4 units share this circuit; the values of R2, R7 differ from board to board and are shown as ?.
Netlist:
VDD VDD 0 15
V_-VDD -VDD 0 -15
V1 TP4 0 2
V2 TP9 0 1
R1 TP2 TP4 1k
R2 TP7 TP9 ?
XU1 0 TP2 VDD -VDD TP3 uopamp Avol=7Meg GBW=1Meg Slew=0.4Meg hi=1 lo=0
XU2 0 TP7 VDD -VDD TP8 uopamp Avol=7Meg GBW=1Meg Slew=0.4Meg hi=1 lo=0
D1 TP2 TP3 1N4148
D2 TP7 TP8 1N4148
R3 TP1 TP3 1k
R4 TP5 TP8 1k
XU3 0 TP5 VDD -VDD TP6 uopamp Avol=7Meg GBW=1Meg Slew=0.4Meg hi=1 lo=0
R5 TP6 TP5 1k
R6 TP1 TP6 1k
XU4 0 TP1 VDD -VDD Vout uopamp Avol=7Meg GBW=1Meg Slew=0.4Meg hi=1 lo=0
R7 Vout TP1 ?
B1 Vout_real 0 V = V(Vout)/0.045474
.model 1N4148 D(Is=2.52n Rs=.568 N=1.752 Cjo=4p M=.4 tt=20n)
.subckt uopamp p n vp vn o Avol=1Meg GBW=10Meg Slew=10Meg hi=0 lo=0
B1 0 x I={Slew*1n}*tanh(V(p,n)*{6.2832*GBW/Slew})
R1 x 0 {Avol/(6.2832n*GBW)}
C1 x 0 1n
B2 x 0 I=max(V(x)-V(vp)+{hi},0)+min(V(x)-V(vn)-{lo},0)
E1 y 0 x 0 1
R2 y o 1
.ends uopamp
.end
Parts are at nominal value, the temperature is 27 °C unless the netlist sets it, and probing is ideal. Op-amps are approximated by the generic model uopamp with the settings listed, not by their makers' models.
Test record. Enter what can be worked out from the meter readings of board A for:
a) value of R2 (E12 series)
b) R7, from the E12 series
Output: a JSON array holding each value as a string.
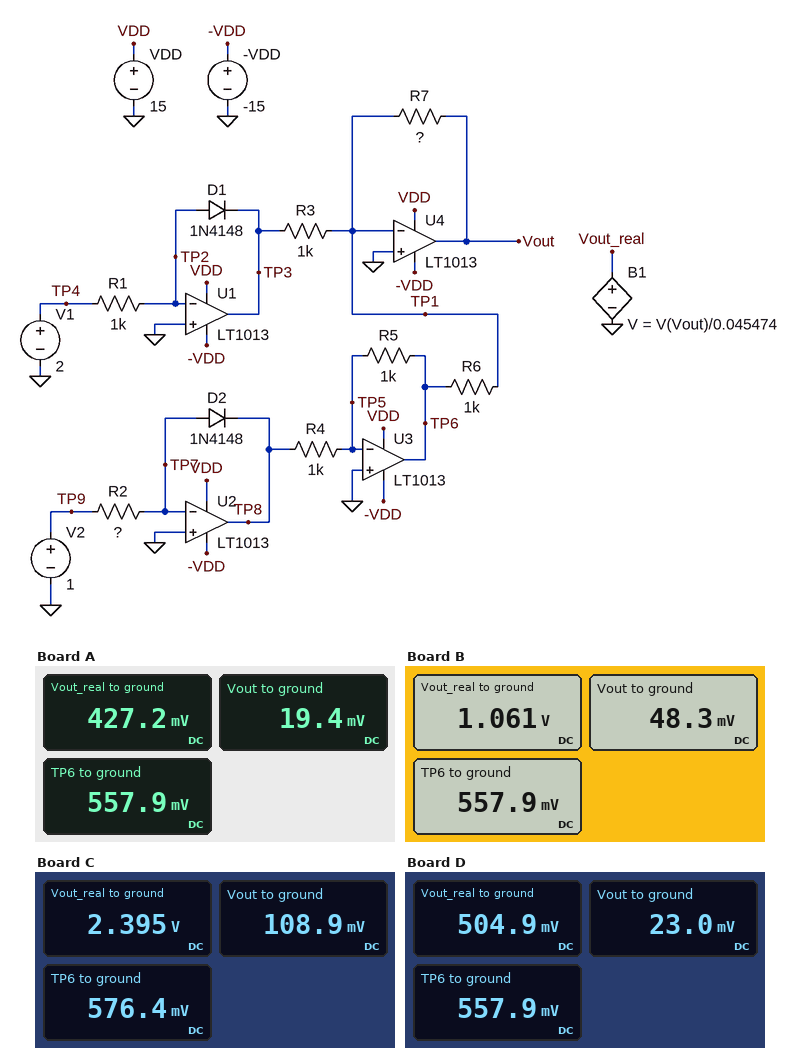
["1.8 kΩ", "330 Ω"]
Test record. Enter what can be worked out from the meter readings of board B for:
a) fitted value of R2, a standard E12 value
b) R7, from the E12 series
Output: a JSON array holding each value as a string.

["1.8 kΩ", "820 Ω"]
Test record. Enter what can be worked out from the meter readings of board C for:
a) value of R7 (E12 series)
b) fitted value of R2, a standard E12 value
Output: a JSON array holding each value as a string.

["2.7 kΩ", "1.2 kΩ"]
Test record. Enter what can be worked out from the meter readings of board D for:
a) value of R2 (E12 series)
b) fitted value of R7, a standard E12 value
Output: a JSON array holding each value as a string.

["1.8 kΩ", "390 Ω"]
